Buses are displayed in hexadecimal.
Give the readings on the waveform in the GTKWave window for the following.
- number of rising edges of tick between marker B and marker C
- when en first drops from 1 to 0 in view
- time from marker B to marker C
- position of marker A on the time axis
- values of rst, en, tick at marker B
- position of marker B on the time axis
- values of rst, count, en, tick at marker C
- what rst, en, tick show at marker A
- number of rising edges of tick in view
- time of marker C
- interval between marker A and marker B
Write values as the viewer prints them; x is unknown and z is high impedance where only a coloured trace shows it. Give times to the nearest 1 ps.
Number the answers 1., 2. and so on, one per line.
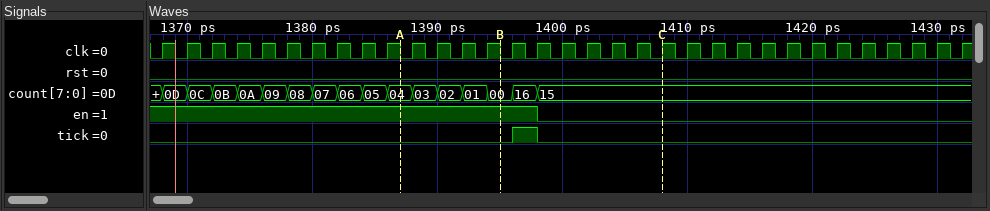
1. 1
2. 1398 ps
3. 13 ps
4. 1387 ps
5. rst=0, en=1, tick=0
6. 1395 ps
7. rst=0, count=15, en=0, tick=0
8. rst=0, en=1, tick=0
9. 1
10. 1408 ps
11. 8 ps
